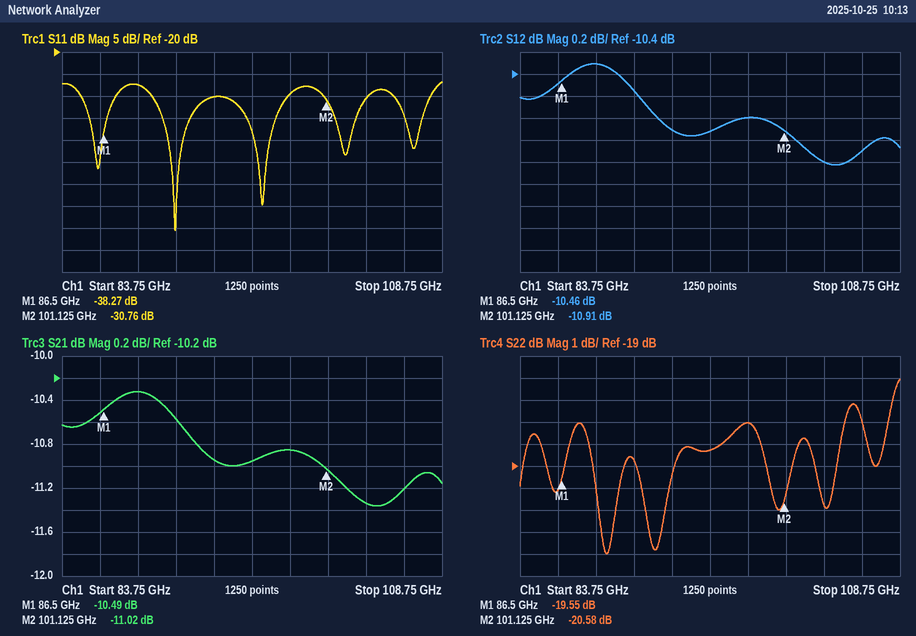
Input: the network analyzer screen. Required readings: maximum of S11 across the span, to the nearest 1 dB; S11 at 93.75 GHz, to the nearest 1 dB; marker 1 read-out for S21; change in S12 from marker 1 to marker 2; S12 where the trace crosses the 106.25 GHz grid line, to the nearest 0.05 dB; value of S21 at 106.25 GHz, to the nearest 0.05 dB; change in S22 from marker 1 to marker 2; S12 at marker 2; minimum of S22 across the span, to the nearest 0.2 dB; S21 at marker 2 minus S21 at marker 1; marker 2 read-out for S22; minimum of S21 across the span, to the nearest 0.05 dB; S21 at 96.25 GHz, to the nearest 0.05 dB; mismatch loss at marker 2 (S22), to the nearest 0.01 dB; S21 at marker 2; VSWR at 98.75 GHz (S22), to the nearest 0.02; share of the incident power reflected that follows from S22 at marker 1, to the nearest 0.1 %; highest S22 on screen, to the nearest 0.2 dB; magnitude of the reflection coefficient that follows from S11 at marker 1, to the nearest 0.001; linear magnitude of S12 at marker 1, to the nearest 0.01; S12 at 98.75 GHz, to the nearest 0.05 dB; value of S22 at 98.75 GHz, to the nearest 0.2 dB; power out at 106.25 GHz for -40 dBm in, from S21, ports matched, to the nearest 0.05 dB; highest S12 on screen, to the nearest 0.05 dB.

-27 dB
-30 dB
-10.49 dB
-0.45 dB
-11.10 dB
-11.20 dB
-1.03 dB
-10.91 dB
-23.0 dB
-0.53 dB
-20.58 dB
-11.35 dB
-10.95 dB
0.04 dB
-11.02 dB
1.32
1.1 %
-15.0 dB
0.012
0.30
-10.80 dB
-17.0 dB
-51.20 dBm
-10.30 dB
